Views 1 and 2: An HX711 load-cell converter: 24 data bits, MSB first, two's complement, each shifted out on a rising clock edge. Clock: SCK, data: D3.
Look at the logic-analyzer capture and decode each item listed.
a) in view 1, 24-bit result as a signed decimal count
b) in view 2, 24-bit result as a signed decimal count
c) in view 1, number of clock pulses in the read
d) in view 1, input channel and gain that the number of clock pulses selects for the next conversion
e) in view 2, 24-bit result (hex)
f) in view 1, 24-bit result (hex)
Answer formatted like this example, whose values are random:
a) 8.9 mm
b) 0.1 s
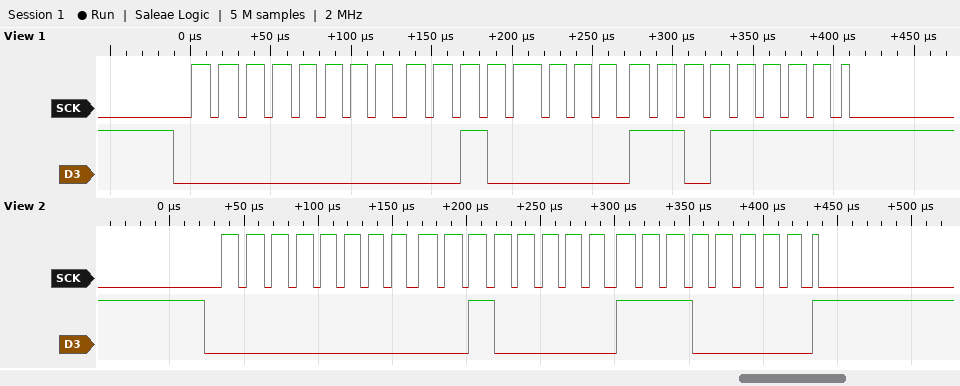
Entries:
a) 8415
b) 8416
c) 25
d) channel A, gain 128
e) 0x0020E0
f) 0x0020DF
